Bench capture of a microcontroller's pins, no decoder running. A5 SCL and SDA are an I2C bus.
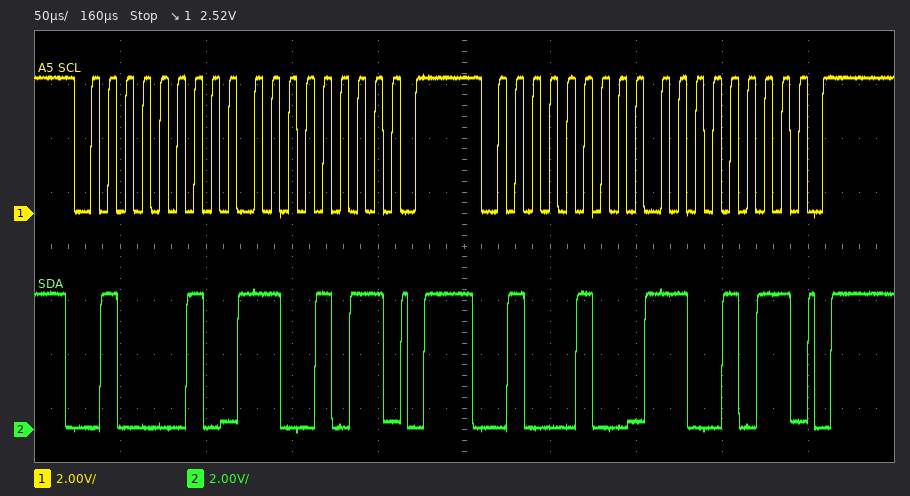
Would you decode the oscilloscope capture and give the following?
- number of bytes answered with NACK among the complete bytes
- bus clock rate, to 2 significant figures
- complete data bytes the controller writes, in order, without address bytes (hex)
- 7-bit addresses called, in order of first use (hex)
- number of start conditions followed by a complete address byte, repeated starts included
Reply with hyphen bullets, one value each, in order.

- 0
- 100 kHz
- CB CB
- 0x21 0x22
- 2
